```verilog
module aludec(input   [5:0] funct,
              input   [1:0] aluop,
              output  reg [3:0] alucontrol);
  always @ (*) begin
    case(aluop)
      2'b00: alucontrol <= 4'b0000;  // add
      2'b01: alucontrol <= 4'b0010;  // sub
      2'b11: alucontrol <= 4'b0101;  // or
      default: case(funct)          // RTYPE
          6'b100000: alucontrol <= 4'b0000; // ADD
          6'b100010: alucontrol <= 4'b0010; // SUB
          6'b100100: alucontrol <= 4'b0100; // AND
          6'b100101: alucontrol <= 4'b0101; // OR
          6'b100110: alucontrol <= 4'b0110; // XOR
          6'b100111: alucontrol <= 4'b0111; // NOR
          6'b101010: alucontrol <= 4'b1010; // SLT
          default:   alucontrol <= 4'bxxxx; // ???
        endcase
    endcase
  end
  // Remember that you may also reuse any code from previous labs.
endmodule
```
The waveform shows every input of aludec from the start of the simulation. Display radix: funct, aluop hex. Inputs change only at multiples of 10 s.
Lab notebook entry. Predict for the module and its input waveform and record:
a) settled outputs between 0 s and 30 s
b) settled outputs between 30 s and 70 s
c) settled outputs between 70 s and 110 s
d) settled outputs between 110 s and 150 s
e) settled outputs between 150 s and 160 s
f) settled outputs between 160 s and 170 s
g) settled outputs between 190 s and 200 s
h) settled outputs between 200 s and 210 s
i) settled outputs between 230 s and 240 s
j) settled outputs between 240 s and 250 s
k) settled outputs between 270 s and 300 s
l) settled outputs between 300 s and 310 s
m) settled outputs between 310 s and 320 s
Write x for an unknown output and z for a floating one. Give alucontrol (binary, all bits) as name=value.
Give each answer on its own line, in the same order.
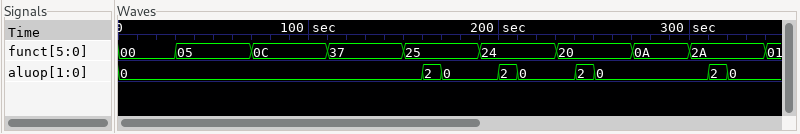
alucontrol=0000
alucontrol=0000
alucontrol=0000
alucontrol=0000
alucontrol=0000
alucontrol=0101
alucontrol=0000
alucontrol=0100
alucontrol=0000
alucontrol=0000
alucontrol=0000
alucontrol=0000
alucontrol=1010
